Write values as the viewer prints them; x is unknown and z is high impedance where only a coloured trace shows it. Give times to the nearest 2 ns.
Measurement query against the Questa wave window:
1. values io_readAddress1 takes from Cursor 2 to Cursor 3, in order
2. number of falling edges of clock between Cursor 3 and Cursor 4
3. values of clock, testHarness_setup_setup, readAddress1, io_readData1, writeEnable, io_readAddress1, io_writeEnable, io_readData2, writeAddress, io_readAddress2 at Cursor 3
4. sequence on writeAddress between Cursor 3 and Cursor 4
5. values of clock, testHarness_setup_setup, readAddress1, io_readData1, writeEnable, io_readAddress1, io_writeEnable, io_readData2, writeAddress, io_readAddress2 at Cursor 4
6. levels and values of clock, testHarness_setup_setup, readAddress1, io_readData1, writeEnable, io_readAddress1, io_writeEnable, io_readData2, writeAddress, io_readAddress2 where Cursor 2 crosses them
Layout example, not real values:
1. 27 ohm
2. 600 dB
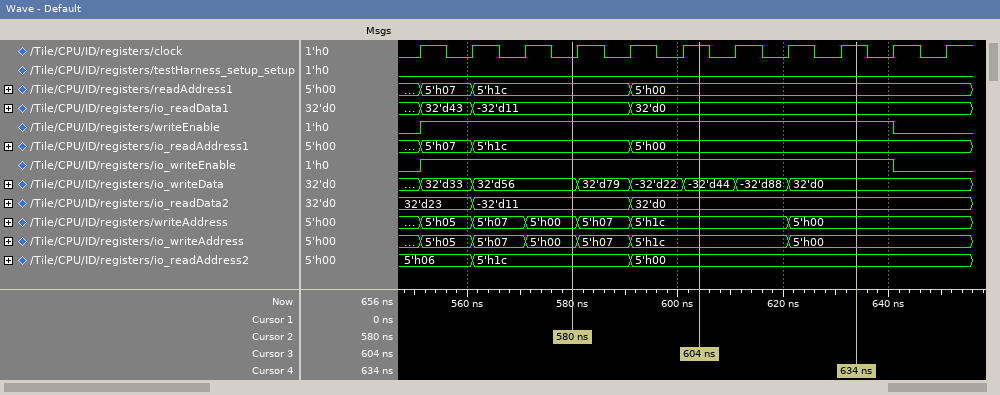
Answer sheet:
1. 5'h1c, 5'h00
2. 3
3. clock=1, testHarness_setup_setup=0, readAddress1=5'h00, io_readData1=32'd0, writeEnable=1, io_readAddress1=5'h00, io_writeEnable=1, io_readData2=32'd0, writeAddress=5'h1c, io_readAddress2=5'h00
4. 5'h1c, 5'h00
5. clock=1, testHarness_setup_setup=0, readAddress1=5'h00, io_readData1=32'd0, writeEnable=1, io_readAddress1=5'h00, io_writeEnable=1, io_readData2=32'd0, writeAddress=5'h00, io_readAddress2=5'h00
6. clock=0, testHarness_setup_setup=0, readAddress1=5'h1c, io_readData1=-32'd11, writeEnable=1, io_readAddress1=5'h1c, io_writeEnable=1, io_readData2=-32'd11, writeAddress=5'h00, io_readAddress2=5'h1c
